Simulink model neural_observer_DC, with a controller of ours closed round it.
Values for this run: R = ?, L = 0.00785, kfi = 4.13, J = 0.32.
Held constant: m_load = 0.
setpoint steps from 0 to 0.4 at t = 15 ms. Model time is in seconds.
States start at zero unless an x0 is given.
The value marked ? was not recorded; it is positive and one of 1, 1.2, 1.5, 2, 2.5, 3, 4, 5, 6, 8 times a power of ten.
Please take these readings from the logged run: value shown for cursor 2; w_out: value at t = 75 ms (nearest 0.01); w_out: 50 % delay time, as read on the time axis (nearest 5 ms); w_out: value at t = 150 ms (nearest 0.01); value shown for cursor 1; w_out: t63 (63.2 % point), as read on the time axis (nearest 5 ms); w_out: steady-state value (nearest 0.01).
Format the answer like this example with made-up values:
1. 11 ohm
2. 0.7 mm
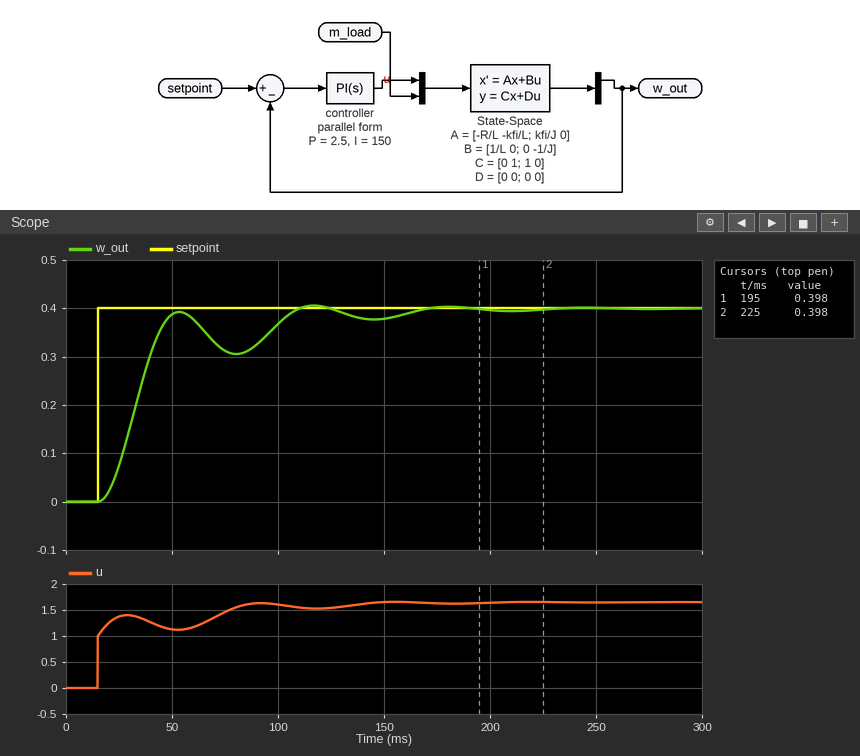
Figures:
1. 0.398
2. 0.31
3. 35 ms
4. 0.38
5. 0.398
6. 35 ms
7. 0.40
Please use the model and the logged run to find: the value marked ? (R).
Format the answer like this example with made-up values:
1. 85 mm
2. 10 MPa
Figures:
1. 0.5
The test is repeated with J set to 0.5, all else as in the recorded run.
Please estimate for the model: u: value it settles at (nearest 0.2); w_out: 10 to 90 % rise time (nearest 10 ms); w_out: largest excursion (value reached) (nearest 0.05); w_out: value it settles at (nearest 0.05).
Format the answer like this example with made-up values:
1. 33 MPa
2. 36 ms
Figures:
1. 1.6
2. 30 ms
3. 0.40
4. 0.40
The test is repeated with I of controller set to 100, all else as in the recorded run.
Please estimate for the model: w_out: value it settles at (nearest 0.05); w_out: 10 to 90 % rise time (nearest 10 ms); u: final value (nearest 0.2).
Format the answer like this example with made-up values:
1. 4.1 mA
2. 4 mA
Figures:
1. 0.40
2. 90 ms
3. 1.6
